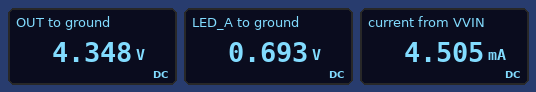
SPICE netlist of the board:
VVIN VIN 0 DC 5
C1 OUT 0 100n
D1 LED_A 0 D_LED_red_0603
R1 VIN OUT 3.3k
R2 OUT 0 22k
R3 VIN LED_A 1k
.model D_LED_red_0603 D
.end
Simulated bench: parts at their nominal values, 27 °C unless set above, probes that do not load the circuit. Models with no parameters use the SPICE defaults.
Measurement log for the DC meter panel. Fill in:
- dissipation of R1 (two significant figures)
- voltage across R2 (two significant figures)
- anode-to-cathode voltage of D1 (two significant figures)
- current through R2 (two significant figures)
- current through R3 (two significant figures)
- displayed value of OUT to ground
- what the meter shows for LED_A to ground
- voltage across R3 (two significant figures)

130 µW
4.3 V
690 mV
200 µA
4.3 mA
4.348 V
0.693 V
4.3 V
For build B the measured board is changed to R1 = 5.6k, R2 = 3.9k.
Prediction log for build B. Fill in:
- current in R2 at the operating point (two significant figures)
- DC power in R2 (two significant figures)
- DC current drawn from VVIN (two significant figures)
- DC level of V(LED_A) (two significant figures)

530 µA
1.1 mW
4.8 mA
690 mV
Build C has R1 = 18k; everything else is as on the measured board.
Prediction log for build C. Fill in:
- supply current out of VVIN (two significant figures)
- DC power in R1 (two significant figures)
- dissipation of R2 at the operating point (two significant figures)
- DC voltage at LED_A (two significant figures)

4.4 mA
280 µW
340 µW
690 mV
